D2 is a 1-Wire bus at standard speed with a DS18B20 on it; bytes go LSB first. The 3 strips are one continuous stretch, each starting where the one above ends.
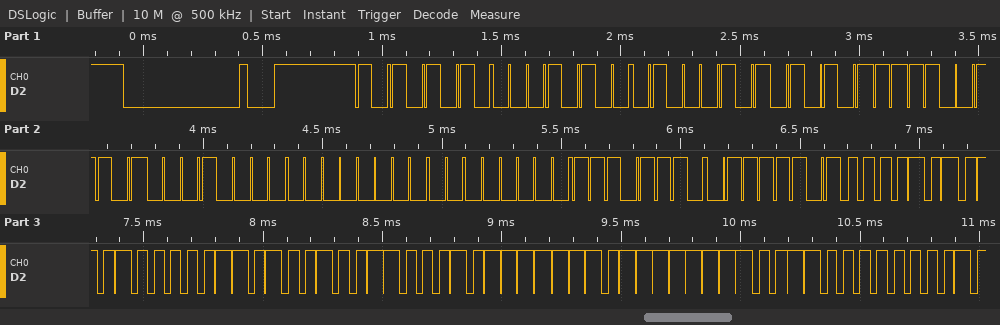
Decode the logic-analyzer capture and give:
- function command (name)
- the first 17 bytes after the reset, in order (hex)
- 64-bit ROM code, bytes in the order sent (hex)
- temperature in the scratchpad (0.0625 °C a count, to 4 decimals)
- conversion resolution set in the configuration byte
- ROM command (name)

Read Scratchpad
55 28 A2 EA B3 08 00 00 77 BE 50 05 4B 46 7F FF 0C
28 A2 EA B3 08 00 00 77
85.0000 °C
12 bits
Match ROM
